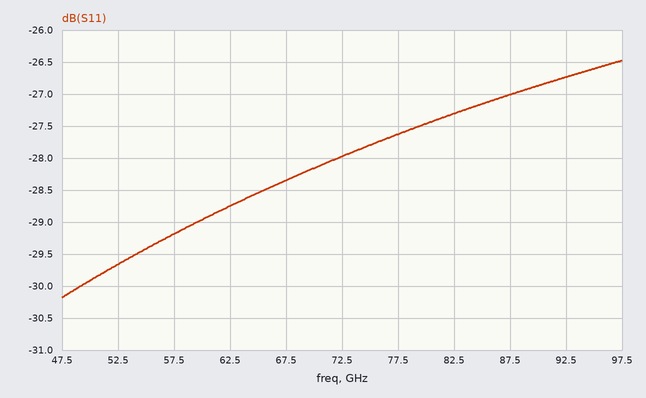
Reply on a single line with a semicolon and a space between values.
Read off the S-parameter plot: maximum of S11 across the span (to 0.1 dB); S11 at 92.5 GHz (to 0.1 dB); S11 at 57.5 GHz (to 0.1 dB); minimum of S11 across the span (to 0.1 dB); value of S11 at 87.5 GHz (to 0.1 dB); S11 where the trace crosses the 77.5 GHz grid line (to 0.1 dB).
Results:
-26.5 dB; -26.7 dB; -29.2 dB; -30.2 dB; -27.0 dB; -27.6 dB
